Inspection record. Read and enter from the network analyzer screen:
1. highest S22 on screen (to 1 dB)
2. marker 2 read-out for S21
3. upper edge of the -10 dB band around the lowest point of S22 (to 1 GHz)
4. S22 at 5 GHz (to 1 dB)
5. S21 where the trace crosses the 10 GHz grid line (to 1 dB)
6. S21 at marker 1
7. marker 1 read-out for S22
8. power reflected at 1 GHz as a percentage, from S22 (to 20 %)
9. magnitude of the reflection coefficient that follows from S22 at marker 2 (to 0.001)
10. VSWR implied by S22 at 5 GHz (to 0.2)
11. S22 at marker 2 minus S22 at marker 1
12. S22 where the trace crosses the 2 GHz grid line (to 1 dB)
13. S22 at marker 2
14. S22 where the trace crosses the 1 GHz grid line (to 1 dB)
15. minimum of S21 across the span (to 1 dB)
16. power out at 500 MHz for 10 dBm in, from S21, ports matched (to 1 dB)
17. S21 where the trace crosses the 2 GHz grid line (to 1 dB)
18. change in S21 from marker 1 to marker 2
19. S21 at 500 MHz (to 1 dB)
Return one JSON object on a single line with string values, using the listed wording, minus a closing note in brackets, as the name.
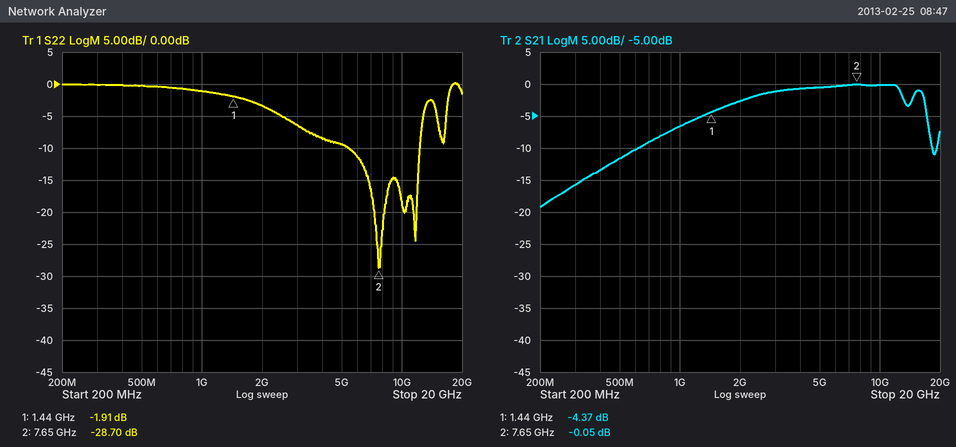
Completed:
{"highest S22 on screen": "0 dB", "marker 2 read-out for S21": "-0.05 dB", "upper edge of the -10 dB band around the lowest point of S22": "12 GHz", "S22 at 5 GHz": "-9 dB", "S21 where the trace crosses the 10 GHz grid line": "0 dB", "S21 at marker 1": "-4.37 dB", "marker 1 read-out for S22": "-1.91 dB", "power reflected at 1 GHz as a percentage, from S22": "80 %", "magnitude of the reflection coefficient that follows from S22 at marker 2": "0.037", "VSWR implied by S22 at 5 GHz": "2.0", "S22 at marker 2 minus S22 at marker 1": "-26.79 dB", "S22 where the trace crosses the 2 GHz grid line": "-3 dB", "S22 at marker 2": "-28.70 dB", "S22 where the trace crosses the 1 GHz grid line": "-1 dB", "minimum of S21 across the span": "-19 dB", "power out at 500 MHz for 10 dBm in, from S21, ports matched": "-2 dBm", "S21 where the trace crosses the 2 GHz grid line": "-3 dB", "change in S21 from marker 1 to marker 2": "4.32 dB", "S21 at 500 MHz": "-12 dB"}
